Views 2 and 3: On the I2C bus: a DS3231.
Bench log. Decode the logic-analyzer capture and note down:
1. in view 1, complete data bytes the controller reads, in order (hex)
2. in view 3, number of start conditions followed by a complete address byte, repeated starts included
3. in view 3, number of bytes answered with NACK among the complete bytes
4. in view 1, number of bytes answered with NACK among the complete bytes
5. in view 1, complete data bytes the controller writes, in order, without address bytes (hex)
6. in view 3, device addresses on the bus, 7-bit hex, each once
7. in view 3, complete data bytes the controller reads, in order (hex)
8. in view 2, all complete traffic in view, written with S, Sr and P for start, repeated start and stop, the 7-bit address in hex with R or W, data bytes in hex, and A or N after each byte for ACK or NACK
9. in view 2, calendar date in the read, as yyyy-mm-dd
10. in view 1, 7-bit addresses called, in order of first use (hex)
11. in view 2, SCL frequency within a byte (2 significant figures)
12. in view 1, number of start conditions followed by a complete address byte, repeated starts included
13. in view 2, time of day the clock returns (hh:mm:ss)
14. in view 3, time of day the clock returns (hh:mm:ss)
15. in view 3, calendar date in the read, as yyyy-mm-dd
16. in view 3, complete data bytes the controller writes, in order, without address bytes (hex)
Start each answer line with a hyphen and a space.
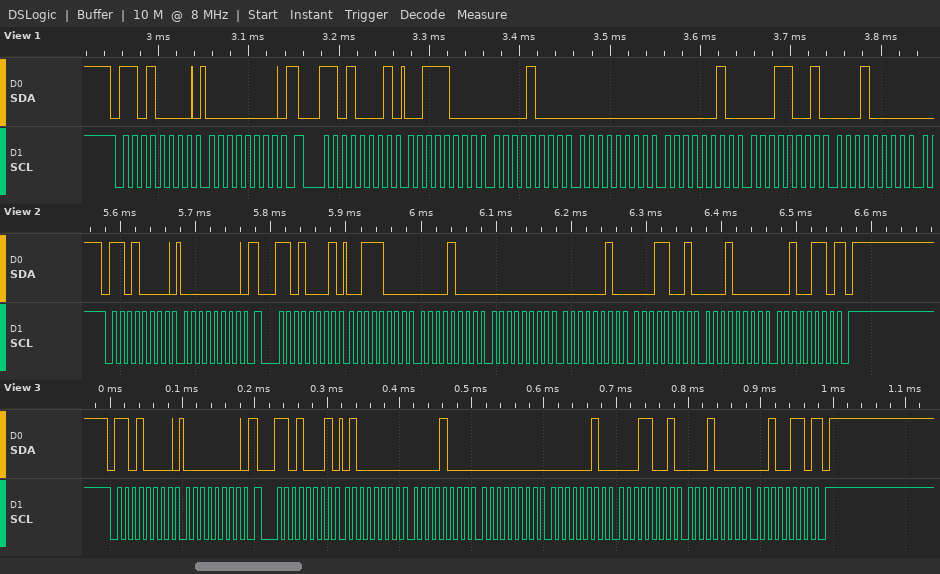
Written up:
- 38 08 00 02 19 10
- 2
- 1
- 0
- 00
- 0x68
- 40 08 00 02 19 10 26
- S 68W A 00 A Sr 68R A 38 A 08 A 00 A 02 A 19 A 10 A 26 N P
- 2026-10-19
- 0x68
- 100 kHz
- 2
- 00:08:38
- 00:08:40
- 2026-10-19
- 00
